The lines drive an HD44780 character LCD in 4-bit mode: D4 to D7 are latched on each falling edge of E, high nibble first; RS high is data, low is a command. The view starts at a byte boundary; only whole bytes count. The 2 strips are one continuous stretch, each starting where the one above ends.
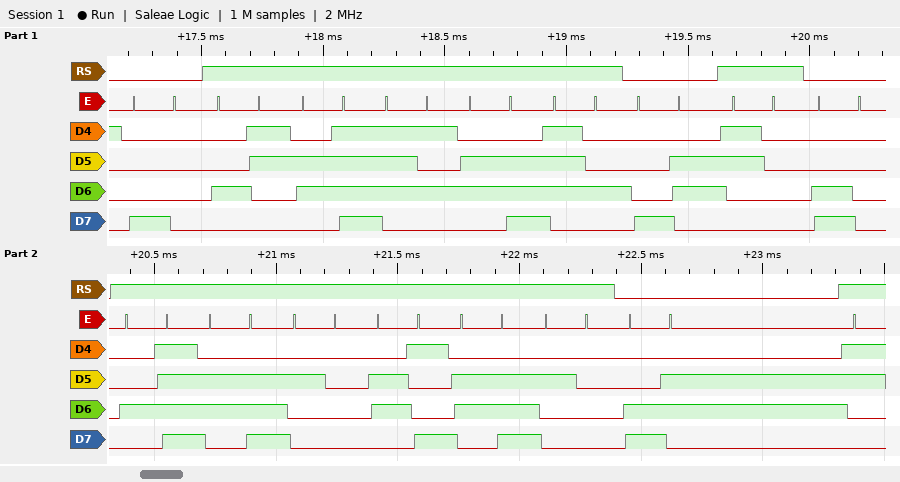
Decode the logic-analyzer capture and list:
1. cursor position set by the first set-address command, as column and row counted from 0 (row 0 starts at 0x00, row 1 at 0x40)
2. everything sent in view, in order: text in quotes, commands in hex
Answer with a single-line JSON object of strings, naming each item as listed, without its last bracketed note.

{"cursor position set by the first set-address command, as column and row counted from 0": "column 0, row 0", "everything sent in view, in order: text in quotes, commands in hex": "0x80 \"Count\" 0x86 \"0\" 0xC0 \"On in \" 0xC6"}
